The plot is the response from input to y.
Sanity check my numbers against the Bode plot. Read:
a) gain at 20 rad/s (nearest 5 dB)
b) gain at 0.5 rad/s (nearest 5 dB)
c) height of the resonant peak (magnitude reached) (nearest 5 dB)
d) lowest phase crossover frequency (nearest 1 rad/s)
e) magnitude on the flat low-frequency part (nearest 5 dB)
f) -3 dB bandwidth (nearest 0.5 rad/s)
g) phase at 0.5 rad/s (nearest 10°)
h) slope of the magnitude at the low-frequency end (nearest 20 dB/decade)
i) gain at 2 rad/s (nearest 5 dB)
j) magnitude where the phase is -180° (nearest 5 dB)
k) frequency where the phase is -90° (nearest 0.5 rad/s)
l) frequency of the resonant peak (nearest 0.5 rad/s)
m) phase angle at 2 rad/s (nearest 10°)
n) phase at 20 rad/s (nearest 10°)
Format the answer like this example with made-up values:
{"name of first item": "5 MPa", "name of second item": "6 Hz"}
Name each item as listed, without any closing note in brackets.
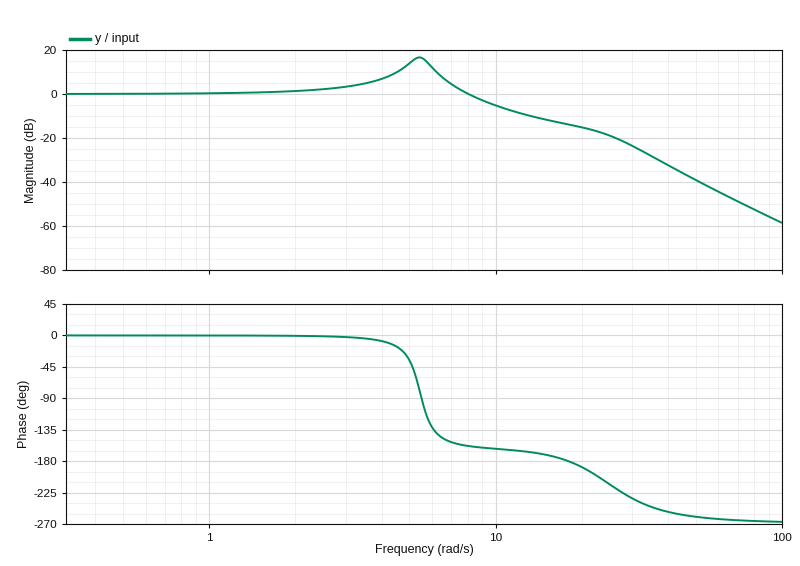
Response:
{"gain at 20 rad/s": "-15 dB", "gain at 0.5 rad/s": "0 dB", "height of the resonant peak (magnitude reached)": "15 dB", "lowest phase crossover frequency": "18 rad/s", "magnitude on the flat low-frequency part": "0 dB", "-3 dB bandwidth": "9.0 rad/s", "phase at 0.5 rad/s": "0°", "slope of the magnitude at the low-frequency end": "0 dB/decade", "gain at 2 rad/s": "0 dB", "magnitude where the phase is -180°": "-15 dB", "frequency where the phase is -90°": "5.5 rad/s", "frequency of the resonant peak": "5.5 rad/s", "phase angle at 2 rad/s": "0°", "phase at 20 rad/s": "-190°"}
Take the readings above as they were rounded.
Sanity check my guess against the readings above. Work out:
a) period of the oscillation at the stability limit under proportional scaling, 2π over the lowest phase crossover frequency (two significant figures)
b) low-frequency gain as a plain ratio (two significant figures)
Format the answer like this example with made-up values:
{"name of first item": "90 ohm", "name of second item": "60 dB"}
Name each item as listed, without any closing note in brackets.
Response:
{"period of the oscillation at the stability limit under proportional scaling, 2π over the lowest phase crossover frequency": "0.35 s", "low-frequency gain as a plain ratio": "1.0"}
